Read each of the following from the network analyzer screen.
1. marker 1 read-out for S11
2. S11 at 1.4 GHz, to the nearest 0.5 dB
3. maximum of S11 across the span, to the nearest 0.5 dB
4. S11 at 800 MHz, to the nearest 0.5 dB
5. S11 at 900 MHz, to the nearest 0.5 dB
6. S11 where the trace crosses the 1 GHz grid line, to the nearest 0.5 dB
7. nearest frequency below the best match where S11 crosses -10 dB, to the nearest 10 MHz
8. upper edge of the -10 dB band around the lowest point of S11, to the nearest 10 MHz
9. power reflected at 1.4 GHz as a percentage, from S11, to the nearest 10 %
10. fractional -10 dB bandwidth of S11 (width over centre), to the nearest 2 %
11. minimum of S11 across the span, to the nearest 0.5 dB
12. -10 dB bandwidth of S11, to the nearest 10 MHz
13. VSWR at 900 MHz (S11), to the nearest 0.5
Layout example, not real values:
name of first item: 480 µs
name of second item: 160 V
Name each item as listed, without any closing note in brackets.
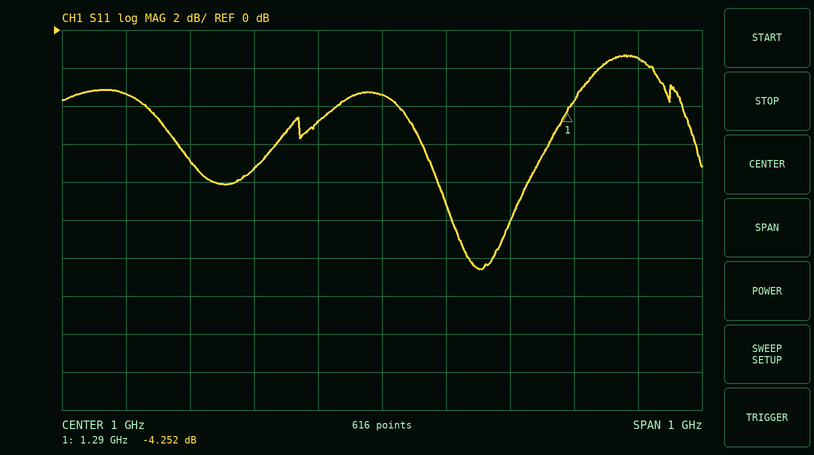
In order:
marker 1 read-out for S11: -4.252 dB
S11 at 1.4 GHz, to the nearest 0.5 dB: -1.5 dB
maximum of S11 across the span, to the nearest 0.5 dB: -1.5 dB
S11 at 800 MHz, to the nearest 0.5 dB: -7.5 dB
S11 at 900 MHz, to the nearest 0.5 dB: -5.0 dB
S11 where the trace crosses the 1 GHz grid line, to the nearest 0.5 dB: -3.5 dB
nearest frequency below the best match where S11 crosses -10 dB, to the nearest 10 MHz: 1.11 GHz
upper edge of the -10 dB band around the lowest point of S11, to the nearest 10 MHz: 1.20 GHz
power reflected at 1.4 GHz as a percentage, from S11, to the nearest 10 %: 70 %
fractional -10 dB bandwidth of S11 (width over centre), to the nearest 2 %: 8 %
minimum of S11 across the span, to the nearest 0.5 dB: -12.5 dB
-10 dB bandwidth of S11, to the nearest 10 MHz: 90 MHz
VSWR at 900 MHz (S11), to the nearest 0.5: 3.5
